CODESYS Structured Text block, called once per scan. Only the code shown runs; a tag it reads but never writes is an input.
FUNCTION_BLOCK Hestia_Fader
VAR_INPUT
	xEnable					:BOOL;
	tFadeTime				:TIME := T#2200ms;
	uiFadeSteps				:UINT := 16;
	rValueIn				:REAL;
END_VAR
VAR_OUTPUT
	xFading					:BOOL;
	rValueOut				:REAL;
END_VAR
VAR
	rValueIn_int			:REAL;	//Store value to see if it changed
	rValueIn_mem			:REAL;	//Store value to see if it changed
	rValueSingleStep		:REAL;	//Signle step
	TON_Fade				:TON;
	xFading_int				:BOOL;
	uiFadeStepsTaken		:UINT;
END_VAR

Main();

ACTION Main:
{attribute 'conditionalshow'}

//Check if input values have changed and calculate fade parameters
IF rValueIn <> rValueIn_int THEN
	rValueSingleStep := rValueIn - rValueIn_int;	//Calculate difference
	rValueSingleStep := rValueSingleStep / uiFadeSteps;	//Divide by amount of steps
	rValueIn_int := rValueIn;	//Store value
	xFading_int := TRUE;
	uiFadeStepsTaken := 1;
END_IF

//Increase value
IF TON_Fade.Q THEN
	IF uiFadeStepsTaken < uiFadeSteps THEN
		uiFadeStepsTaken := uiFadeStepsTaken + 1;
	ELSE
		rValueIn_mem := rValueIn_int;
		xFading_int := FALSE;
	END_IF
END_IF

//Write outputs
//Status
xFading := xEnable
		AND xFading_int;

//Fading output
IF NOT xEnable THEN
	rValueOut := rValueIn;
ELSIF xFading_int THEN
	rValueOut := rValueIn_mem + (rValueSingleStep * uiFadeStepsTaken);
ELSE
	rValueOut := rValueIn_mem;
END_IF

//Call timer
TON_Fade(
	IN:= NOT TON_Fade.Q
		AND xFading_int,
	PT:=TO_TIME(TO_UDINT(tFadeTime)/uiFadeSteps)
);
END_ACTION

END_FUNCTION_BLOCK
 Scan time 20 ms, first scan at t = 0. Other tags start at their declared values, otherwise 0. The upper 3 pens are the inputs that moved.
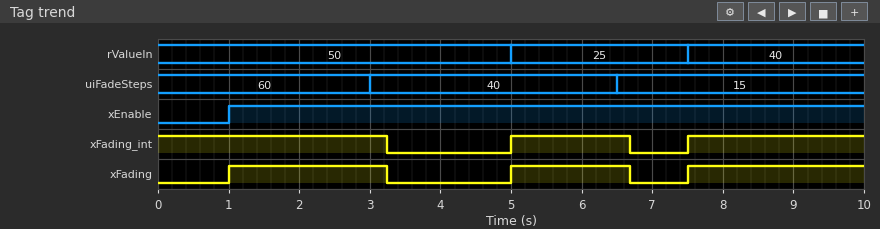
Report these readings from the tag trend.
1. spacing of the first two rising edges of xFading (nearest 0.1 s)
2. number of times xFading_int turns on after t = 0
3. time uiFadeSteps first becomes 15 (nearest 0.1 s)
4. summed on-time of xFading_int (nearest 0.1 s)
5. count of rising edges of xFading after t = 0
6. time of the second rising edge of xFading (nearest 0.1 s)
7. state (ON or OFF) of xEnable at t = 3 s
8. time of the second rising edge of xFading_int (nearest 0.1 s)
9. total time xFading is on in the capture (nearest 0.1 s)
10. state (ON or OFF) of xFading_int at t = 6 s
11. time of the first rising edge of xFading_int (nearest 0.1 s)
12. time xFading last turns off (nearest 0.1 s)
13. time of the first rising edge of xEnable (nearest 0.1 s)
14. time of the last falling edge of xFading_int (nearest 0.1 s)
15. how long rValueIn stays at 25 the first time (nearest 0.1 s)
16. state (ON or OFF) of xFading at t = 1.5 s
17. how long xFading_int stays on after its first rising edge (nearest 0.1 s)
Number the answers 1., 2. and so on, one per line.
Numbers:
1. 4.0 s
2. 2
3. 6.5 s
4. 7.4 s
5. 3
6. 5.0 s
7. ON
8. 7.5 s
9. 6.4 s
10. ON
11. 5.0 s
12. 6.7 s
13. 1.0 s
14. 6.7 s
15. 2.5 s
16. ON
17. 1.7 s
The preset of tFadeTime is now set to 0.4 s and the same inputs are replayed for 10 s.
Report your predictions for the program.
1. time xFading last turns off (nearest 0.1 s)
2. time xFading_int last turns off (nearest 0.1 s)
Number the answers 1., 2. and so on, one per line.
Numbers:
1. 8.7 s
2. 8.7 s
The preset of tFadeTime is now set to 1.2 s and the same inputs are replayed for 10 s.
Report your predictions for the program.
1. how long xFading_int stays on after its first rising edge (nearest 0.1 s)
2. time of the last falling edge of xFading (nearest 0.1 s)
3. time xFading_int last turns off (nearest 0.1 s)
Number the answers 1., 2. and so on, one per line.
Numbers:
1. 1.5 s
2. 9.3 s
3. 9.3 s
